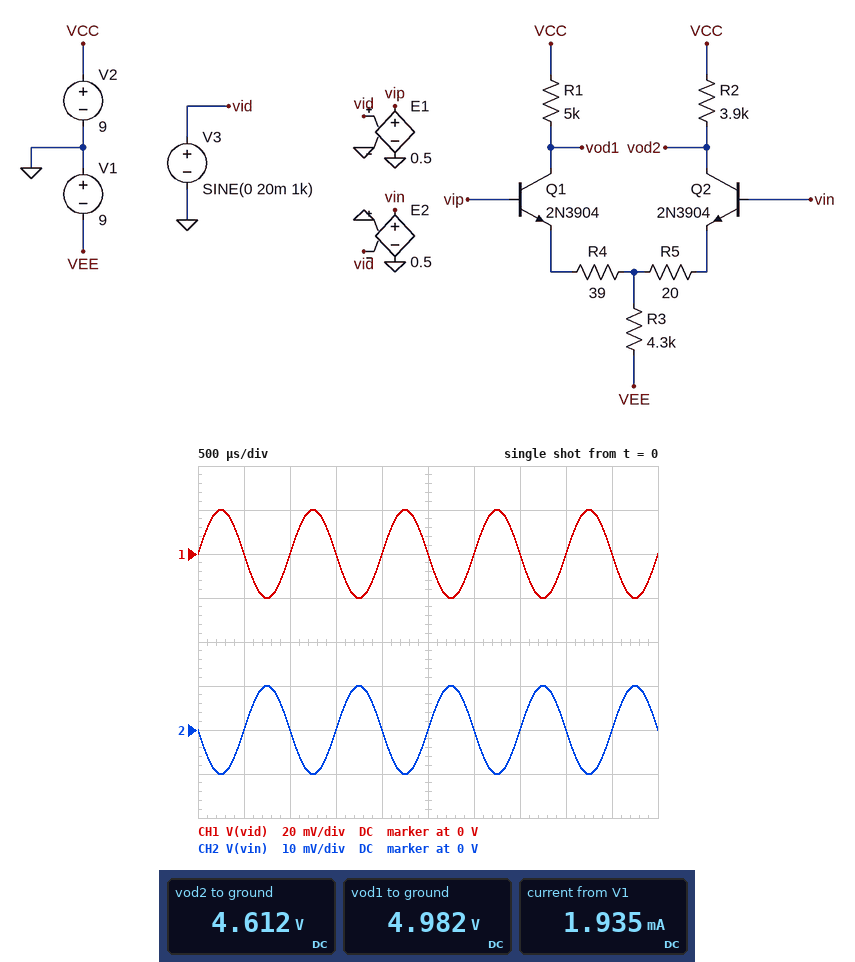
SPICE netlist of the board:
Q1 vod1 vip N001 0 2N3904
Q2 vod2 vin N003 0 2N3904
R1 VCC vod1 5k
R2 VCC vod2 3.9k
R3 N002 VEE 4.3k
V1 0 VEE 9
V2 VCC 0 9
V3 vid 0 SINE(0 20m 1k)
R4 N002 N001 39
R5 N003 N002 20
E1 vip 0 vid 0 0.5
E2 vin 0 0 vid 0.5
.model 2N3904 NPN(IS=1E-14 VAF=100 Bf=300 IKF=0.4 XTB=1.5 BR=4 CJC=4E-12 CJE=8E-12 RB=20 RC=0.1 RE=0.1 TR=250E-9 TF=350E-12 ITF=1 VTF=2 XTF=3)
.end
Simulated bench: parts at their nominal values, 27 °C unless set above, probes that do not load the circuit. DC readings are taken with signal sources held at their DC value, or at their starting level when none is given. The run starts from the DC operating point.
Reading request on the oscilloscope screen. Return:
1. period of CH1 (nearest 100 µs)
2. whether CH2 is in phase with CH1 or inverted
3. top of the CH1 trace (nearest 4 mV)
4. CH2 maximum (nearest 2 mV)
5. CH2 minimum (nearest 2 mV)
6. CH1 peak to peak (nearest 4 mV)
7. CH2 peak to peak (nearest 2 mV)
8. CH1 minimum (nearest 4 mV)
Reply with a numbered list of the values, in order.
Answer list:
1. 1.0 ms
2. inverted
3. 20 mV
4. 10 mV
5. -10 mV
6. 40 mV
7. 20 mV
8. -20 mV
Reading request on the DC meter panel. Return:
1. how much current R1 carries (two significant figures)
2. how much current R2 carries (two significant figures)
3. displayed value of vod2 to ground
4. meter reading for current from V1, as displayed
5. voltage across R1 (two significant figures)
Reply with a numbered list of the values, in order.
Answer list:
1. 800 µA
2. 1.1 mA
3. 4.612 V
4. 1.935 mA
5. 4.0 V
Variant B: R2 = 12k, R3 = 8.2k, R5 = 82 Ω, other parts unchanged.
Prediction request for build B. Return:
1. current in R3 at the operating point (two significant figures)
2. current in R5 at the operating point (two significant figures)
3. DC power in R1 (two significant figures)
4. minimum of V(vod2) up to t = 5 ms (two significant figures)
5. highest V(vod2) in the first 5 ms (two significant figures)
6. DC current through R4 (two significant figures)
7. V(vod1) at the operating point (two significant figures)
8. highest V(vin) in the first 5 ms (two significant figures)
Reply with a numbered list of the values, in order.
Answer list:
1. 1.0 mA
2. 410 µA
3. 1.8 mW
4. 3.1 V
5. 5.1 V
6. 610 µA
7. 6.0 V
8. 10 mV
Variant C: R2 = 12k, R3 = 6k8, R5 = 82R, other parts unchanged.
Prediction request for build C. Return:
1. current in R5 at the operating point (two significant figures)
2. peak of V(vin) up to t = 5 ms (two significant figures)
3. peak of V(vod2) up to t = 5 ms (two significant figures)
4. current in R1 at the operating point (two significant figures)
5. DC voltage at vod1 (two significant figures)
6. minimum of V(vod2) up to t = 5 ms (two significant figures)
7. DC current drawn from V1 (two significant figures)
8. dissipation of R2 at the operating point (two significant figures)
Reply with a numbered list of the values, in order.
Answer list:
1. 480 µA
2. 10 mV
3. 4.3 V
4. 740 µA
5. 5.3 V
6. 2.1 V
7. 1.2 mA
8. 2.8 mW
